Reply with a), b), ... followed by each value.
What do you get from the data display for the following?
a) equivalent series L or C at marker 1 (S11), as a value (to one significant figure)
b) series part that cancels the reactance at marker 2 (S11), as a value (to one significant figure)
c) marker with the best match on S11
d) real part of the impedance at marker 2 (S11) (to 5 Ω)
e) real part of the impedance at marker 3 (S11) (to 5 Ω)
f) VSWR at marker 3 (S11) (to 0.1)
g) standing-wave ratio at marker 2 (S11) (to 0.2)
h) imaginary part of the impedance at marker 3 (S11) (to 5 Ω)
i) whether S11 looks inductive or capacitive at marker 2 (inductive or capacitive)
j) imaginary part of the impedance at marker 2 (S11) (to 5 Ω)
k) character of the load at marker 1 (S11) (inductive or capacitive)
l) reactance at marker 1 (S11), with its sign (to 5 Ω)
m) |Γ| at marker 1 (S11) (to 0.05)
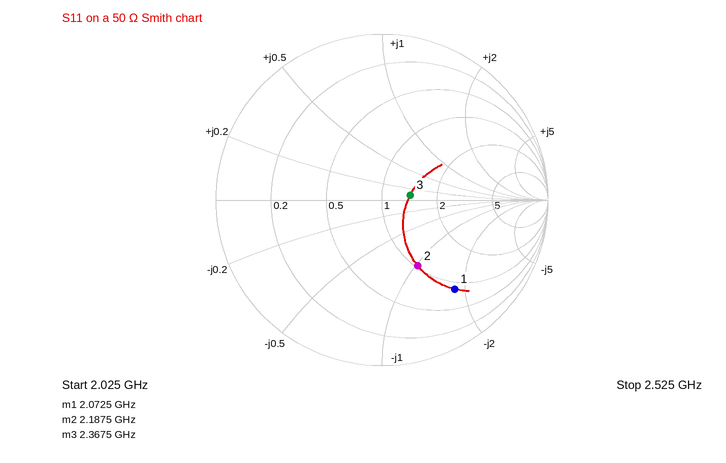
a) 900 fF
b) 4 nH
c) marker 3
d) 50 Ω
e) 70 Ω
f) 1.4
g) 2.6
h) +5 Ω
i) capacitive
j) -50 Ω
k) capacitive
l) -90 Ω
m) 0.70
